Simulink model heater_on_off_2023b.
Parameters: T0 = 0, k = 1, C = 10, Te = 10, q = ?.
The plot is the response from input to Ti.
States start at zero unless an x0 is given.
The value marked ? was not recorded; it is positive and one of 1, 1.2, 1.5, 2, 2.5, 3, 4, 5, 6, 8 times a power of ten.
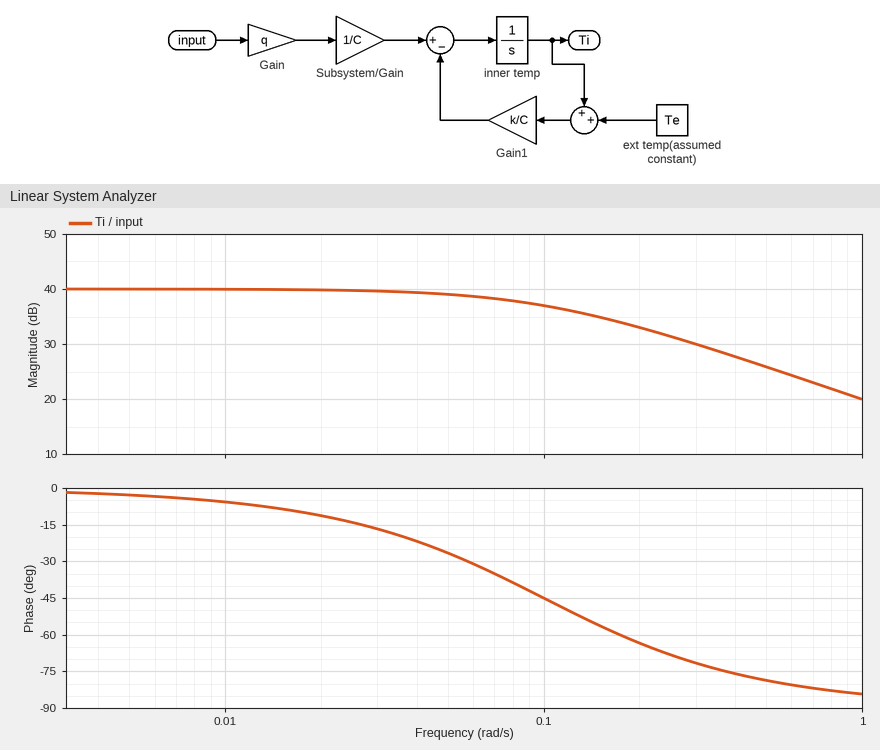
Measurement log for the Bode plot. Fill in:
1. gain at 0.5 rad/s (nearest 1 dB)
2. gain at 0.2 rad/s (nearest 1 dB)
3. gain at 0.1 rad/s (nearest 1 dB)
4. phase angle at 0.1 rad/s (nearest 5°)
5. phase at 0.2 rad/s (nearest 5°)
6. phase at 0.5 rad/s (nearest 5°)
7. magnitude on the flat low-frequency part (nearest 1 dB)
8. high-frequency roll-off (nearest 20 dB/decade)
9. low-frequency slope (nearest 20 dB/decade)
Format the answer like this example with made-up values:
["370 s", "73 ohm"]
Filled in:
["26 dB", "33 dB", "37 dB", "-45°", "-65°", "-80°", "40 dB", "-20 dB/decade", "0 dB/decade"]
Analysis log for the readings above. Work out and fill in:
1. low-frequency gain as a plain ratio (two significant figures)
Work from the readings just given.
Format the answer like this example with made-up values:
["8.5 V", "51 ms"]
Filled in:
["100"]
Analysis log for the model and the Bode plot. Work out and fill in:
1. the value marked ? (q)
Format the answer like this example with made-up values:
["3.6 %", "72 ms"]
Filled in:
["100"]
